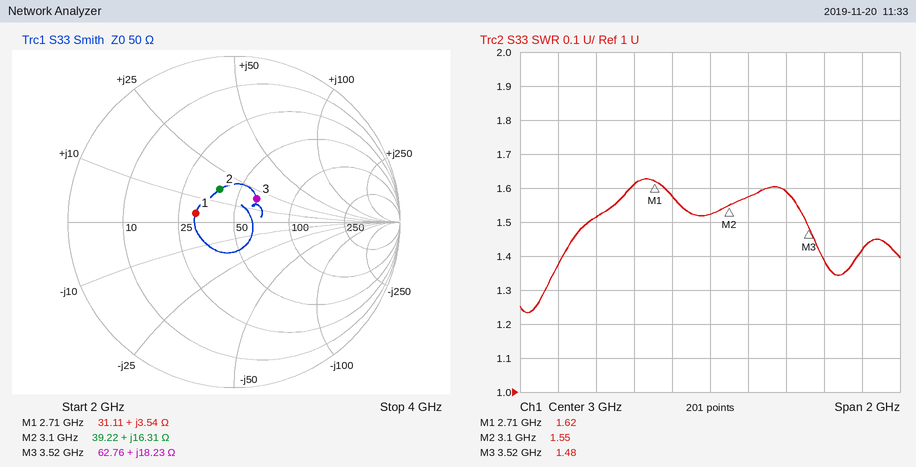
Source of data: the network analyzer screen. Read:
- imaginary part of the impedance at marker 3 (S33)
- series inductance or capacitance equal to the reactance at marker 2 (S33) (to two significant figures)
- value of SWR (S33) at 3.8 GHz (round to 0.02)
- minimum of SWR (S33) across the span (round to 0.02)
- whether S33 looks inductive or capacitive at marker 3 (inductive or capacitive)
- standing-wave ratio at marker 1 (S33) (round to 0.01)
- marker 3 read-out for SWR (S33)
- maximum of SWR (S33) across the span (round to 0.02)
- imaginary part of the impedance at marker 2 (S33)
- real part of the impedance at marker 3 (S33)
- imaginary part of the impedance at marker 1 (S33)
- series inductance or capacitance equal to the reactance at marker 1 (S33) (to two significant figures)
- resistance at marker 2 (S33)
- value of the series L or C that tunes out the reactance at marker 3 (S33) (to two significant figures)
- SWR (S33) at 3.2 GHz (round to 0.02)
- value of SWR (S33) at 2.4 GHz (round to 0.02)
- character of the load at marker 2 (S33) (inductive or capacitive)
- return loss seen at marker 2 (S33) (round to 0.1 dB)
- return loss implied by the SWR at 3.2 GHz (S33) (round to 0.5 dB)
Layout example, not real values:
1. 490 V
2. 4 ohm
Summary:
1. +18.23 Ω
2. 840 pH
3. 1.42
4. 1.24
5. inductive
6. 1.62
7. 1.48
8. 1.62
9. +16.31 Ω
10. 62.76 Ω
11. +3.54 Ω
12. 210 pH
13. 39.22 Ω
14. 2.5 pF
15. 1.58
16. 1.52
17. inductive
18. 13.3 dB
19. 13.0 dB
